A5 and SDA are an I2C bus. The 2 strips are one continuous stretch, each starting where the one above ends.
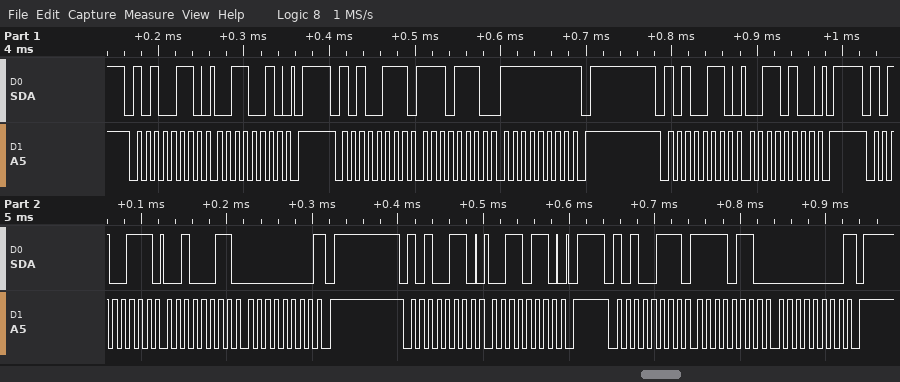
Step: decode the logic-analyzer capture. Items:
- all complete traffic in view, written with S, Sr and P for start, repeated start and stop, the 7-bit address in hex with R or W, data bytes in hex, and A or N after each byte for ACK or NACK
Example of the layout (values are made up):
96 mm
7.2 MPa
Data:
S 53W A 32 A P S 53R A EE A FF N P S 53W A 34 A P S 53R A 23 A 00 N P S 53W A 36 A P S 53R A F6 A 00 N P
